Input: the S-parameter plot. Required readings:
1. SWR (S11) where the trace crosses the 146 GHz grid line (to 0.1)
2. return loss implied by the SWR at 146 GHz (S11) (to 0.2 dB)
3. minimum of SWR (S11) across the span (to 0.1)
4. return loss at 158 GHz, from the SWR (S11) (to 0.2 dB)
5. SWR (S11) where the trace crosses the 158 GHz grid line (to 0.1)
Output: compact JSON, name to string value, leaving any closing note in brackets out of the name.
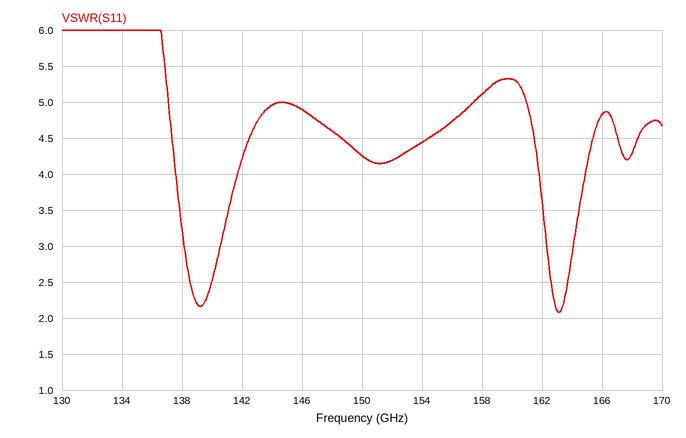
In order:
{"SWR (S11) where the trace crosses the 146 GHz grid line": "4.9", "return loss implied by the SWR at 146 GHz (S11)": "3.6 dB", "minimum of SWR (S11) across the span": "2.1", "return loss at 158 GHz, from the SWR (S11)": "3.4 dB", "SWR (S11) where the trace crosses the 158 GHz grid line": "5.1"}
